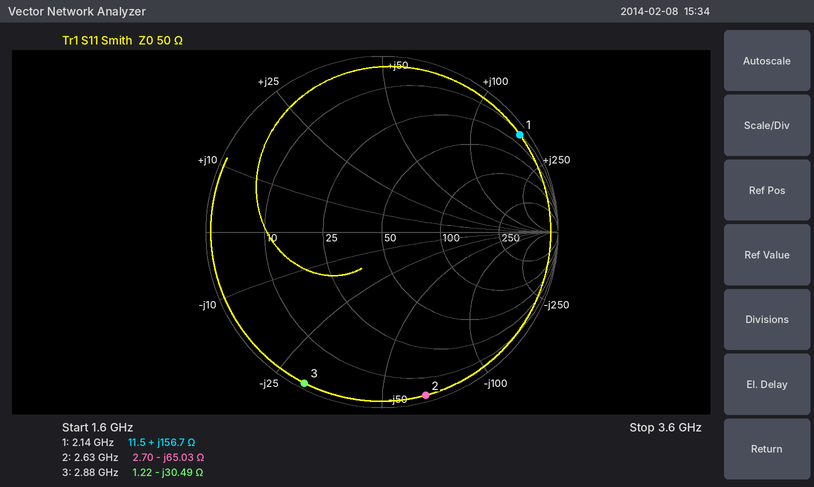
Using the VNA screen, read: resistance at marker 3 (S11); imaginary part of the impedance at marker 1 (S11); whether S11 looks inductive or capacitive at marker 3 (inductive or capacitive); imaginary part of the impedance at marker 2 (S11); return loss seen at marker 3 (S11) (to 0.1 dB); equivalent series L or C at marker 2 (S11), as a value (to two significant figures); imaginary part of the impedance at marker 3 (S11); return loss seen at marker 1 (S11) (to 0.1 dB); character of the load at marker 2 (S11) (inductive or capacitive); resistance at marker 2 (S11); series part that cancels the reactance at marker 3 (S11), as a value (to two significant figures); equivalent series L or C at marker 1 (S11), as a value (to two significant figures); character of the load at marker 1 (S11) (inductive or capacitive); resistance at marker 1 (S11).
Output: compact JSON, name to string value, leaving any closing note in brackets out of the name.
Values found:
{"resistance at marker 3": "1.22 Ω", "imaginary part of the impedance at marker 1": "+156.7 Ω", "whether S11 looks inductive or capacitive at marker 3": "capacitive", "imaginary part of the impedance at marker 2": "-65.03 Ω", "return loss seen at marker 3 (S11)": "0.3 dB", "equivalent series L or C at marker 2 (S11), as a value": "930 fF", "imaginary part of the impedance at marker 3": "-30.49 Ω", "return loss seen at marker 1 (S11)": "0.4 dB", "character of the load at marker 2 (S11)": "capacitive", "resistance at marker 2": "2.70 Ω", "series part that cancels the reactance at marker 3 (S11), as a value": "1.7 nH", "equivalent series L or C at marker 1 (S11), as a value": "12 nH", "character of the load at marker 1 (S11)": "inductive", "resistance at marker 1": "11.5 Ω"}
